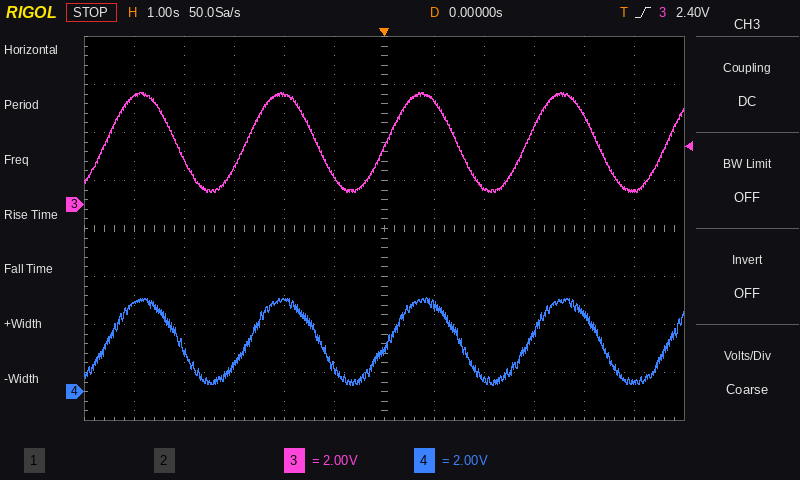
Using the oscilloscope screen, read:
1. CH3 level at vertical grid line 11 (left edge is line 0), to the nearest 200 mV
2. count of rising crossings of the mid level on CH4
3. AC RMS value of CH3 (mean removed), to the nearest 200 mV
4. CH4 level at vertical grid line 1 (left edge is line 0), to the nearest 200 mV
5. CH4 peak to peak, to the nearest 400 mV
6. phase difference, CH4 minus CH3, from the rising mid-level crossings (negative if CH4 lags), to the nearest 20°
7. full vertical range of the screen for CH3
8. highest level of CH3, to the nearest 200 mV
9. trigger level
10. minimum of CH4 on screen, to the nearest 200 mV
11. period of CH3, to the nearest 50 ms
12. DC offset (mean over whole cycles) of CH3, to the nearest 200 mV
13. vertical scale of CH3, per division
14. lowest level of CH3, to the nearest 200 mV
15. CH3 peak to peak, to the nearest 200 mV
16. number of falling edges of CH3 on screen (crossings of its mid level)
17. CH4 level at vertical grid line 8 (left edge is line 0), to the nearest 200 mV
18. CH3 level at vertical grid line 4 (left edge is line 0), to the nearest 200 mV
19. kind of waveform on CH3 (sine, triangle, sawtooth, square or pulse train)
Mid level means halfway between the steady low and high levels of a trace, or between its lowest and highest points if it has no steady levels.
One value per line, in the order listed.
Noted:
600 mV
5
1.4 V
3.6 V
3.6 V
0°
16 V
4.6 V
2.40 V
200 mV
2.80 s
2.6 V
2 V
400 mV
4.2 V
4
600 mV
4.6 V
sine
